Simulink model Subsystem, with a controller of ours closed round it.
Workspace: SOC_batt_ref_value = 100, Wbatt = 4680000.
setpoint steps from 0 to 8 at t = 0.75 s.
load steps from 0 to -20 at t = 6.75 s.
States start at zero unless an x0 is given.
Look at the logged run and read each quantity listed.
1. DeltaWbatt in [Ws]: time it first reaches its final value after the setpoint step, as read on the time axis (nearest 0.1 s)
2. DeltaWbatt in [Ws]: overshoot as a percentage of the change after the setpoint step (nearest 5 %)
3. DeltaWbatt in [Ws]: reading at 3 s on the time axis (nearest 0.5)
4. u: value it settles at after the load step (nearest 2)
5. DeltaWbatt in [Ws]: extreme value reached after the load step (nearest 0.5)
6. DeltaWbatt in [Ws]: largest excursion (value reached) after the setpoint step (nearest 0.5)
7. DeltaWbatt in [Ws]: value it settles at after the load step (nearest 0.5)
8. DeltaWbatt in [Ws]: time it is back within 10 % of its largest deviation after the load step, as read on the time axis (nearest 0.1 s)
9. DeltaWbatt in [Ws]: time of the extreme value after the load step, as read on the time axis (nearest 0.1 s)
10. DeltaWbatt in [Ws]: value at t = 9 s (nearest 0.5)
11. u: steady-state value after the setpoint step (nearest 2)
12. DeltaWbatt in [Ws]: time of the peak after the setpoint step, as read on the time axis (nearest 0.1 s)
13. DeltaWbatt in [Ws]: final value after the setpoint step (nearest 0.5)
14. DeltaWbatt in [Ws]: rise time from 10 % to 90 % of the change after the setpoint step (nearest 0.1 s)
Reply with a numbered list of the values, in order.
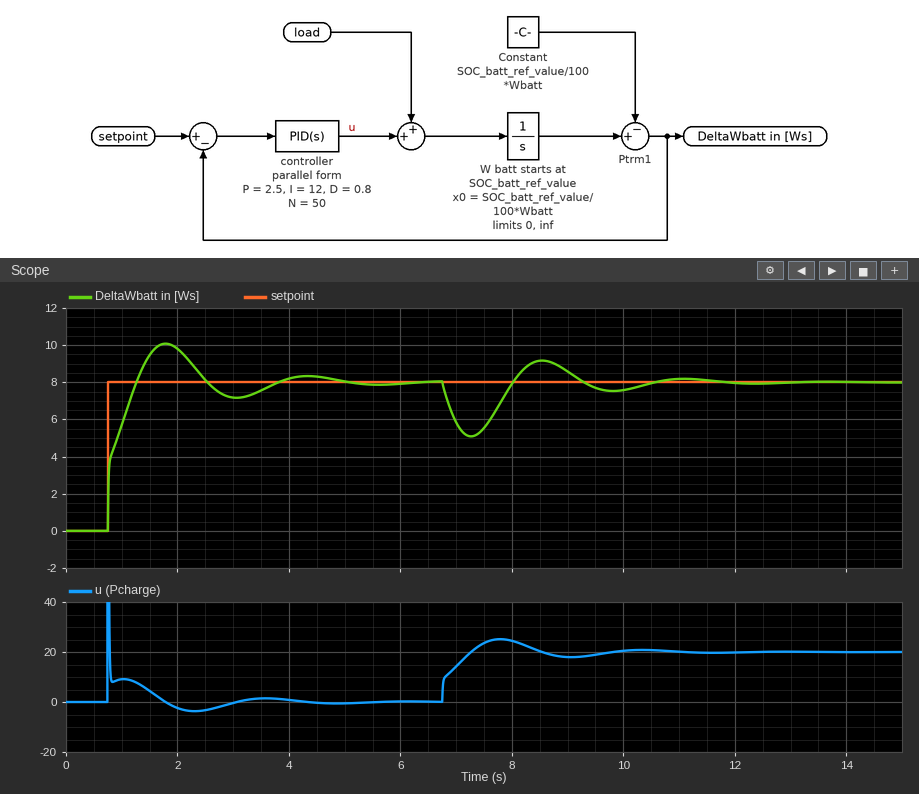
1. 1.3 s
2. 25 %
3. 7.0
4. 20
5. 5.0
6. 10.0
7. 8.0
8. 10.2 s
9. 7.3 s
10. 8.5
11. 0
12. 1.8 s
13. 8.0
14. 0.4 s
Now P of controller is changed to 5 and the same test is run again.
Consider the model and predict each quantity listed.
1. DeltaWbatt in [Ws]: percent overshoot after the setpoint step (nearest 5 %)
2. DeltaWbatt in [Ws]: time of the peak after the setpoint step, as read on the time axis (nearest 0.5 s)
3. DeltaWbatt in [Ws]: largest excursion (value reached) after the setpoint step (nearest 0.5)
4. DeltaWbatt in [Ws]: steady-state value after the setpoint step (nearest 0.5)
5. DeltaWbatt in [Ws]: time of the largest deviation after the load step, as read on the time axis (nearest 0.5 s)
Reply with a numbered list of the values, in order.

1. 15 %
2. 1.5 s
3. 9.0
4. 8.0
5. 7.0 s
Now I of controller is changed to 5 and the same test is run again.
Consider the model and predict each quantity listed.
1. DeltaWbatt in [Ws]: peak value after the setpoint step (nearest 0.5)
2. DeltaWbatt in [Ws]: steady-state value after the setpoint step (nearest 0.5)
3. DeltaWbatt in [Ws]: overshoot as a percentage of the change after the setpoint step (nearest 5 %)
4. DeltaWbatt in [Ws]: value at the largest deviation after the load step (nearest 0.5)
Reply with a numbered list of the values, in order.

1. 9.5
2. 8.0
3. 20 %
4. 4.0
